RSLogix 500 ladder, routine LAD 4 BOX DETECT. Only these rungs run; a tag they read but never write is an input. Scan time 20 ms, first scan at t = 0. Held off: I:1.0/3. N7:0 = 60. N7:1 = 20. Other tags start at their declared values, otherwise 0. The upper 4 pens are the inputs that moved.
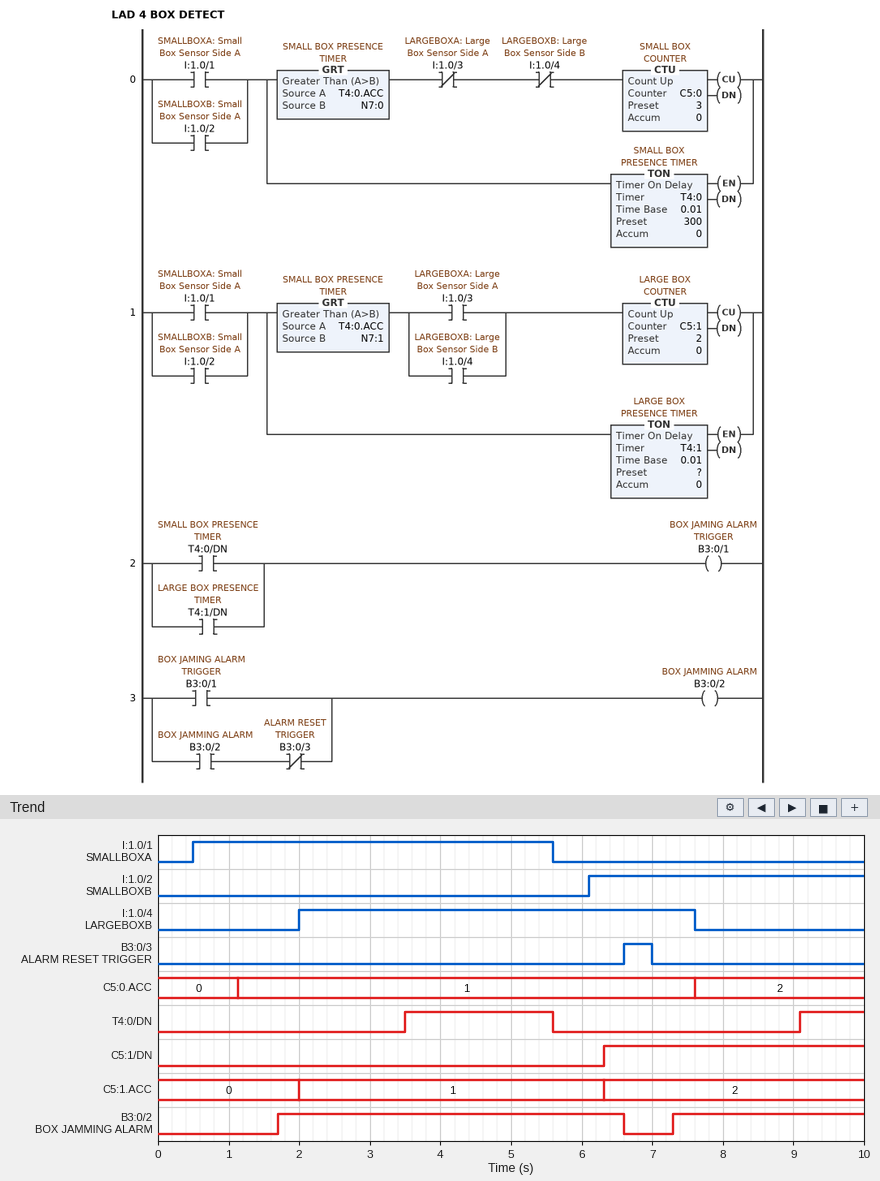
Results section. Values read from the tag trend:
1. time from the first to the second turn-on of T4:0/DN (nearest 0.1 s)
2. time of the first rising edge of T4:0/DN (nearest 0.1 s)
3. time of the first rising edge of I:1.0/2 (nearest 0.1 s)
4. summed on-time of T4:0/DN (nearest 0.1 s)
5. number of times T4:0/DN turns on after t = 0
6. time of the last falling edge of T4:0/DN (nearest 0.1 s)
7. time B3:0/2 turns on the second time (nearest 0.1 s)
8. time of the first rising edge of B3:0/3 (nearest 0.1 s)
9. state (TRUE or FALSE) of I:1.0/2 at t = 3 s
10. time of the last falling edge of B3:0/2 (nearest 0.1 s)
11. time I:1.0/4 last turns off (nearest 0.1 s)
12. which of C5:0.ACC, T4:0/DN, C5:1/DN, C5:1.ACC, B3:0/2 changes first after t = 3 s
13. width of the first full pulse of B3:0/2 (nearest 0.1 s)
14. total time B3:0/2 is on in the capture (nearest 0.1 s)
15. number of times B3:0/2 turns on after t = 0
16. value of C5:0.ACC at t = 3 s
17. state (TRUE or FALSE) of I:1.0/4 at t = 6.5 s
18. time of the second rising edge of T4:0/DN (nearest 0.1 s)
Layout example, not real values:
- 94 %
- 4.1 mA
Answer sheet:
- 5.6 s
- 3.5 s
- 6.1 s
- 3.0 s
- 2
- 5.6 s
- 7.3 s
- 6.6 s
- FALSE
- 6.6 s
- 7.6 s
- T4:0/DN
- 4.9 s
- 7.6 s
- 2
- 1
- TRUE
- 9.1 s
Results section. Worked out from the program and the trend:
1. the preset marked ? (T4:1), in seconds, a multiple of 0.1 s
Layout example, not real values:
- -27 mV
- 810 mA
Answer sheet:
- 1.2 s
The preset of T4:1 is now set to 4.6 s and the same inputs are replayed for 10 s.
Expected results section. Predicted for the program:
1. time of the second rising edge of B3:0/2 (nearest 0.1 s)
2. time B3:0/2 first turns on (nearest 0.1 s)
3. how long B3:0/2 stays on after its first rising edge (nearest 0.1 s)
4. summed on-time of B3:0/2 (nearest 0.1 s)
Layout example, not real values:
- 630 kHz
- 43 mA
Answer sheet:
- 9.1 s
- 3.5 s
- 3.1 s
- 4.0 s
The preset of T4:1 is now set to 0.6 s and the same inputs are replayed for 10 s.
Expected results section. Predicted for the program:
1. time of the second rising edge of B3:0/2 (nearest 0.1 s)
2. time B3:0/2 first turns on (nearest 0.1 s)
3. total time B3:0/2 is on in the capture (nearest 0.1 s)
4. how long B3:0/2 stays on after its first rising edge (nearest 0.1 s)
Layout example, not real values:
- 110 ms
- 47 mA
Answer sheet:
- 6.7 s
- 1.1 s
- 8.8 s
- 5.5 s
